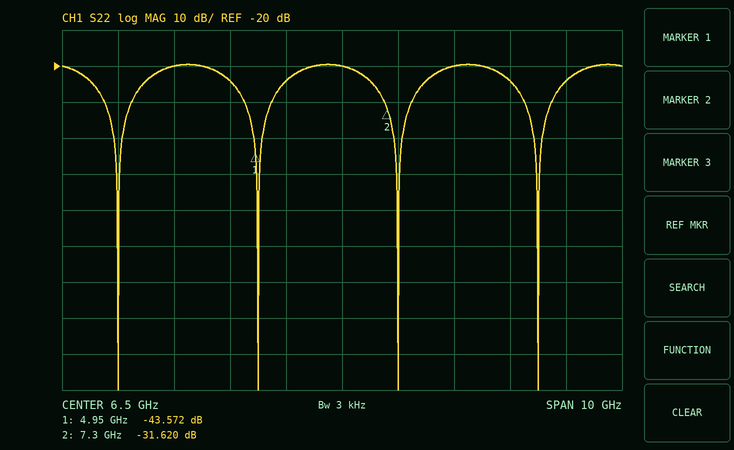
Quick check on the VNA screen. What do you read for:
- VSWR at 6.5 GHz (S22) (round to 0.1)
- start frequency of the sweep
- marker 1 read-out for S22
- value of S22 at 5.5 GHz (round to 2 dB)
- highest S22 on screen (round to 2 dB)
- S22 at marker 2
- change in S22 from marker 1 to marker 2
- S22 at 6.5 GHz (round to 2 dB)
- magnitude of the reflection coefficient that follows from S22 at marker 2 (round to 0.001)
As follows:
1.2
1.5 GHz
-43.572 dB
-24 dB
-20 dB
-31.620 dB
11.952 dB
-20 dB
0.026
